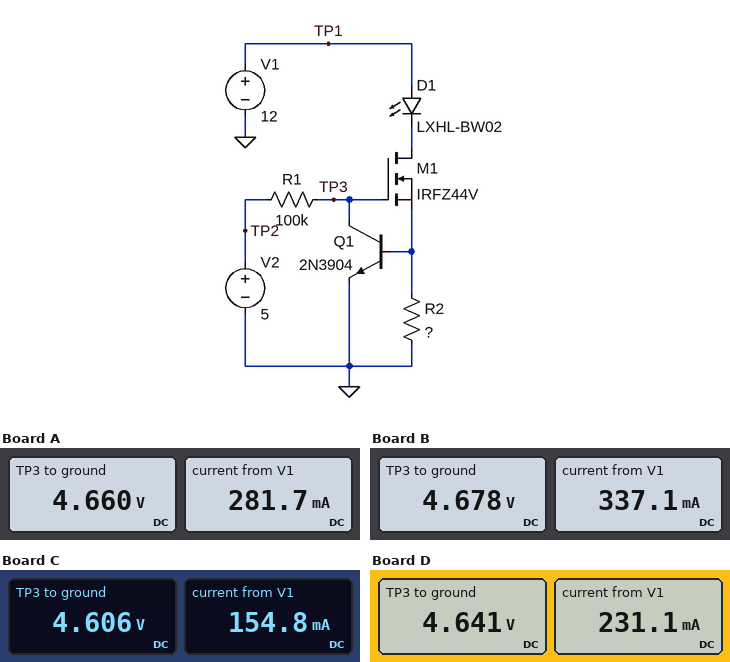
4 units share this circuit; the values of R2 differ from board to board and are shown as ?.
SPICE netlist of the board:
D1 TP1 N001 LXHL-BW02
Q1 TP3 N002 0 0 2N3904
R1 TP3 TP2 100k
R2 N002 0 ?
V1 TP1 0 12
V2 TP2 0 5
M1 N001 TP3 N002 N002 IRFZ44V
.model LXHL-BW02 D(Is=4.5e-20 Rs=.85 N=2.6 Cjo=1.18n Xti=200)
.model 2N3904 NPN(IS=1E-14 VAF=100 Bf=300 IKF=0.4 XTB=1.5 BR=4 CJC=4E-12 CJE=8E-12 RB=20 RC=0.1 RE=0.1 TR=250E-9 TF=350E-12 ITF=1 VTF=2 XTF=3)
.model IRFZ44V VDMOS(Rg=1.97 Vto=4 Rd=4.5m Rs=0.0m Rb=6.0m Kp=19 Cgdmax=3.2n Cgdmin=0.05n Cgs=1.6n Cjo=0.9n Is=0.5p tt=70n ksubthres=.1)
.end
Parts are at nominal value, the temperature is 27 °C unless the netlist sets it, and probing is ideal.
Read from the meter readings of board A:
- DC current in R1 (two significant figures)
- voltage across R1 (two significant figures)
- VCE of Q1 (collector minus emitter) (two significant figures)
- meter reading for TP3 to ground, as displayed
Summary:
3.4 µA
340 mV
4.7 V
4.660 V
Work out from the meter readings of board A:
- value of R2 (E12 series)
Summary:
1.8 Ω
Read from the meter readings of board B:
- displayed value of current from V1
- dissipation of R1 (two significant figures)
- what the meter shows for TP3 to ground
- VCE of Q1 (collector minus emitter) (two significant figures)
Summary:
337.1 mA
1.0 µW
4.678 V
4.7 V
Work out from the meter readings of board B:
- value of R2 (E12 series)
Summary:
1.5 Ω
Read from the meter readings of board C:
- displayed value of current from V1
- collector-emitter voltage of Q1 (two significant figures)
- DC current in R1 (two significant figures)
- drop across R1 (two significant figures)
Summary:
154.8 mA
4.6 V
3.9 µA
390 mV
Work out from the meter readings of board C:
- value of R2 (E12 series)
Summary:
3.3 Ω
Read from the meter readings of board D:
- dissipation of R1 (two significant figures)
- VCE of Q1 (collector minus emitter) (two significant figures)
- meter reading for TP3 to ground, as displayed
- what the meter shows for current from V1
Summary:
1.3 µW
4.6 V
4.641 V
231.1 mA
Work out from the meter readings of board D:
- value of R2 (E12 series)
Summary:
2.2 Ω
